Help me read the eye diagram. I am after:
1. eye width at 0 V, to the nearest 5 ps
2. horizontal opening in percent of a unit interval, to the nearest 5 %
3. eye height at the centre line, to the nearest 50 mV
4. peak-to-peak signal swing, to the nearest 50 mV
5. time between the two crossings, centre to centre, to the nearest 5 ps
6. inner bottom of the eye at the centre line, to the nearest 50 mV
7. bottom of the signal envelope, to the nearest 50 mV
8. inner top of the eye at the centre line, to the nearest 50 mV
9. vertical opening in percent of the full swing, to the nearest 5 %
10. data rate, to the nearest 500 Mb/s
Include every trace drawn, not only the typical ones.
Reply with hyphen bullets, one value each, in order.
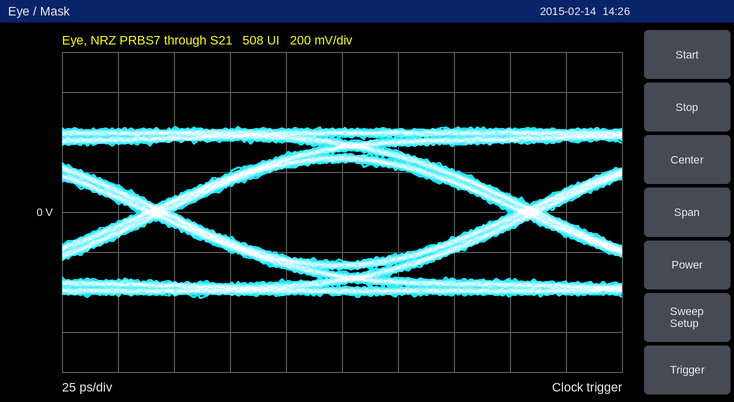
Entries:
- 150 ps
- 90 %
- 500 mV
- 850 mV
- 165 ps
- -250 mV
- -450 mV
- 250 mV
- 60 %
- 6.0 Gb/s
